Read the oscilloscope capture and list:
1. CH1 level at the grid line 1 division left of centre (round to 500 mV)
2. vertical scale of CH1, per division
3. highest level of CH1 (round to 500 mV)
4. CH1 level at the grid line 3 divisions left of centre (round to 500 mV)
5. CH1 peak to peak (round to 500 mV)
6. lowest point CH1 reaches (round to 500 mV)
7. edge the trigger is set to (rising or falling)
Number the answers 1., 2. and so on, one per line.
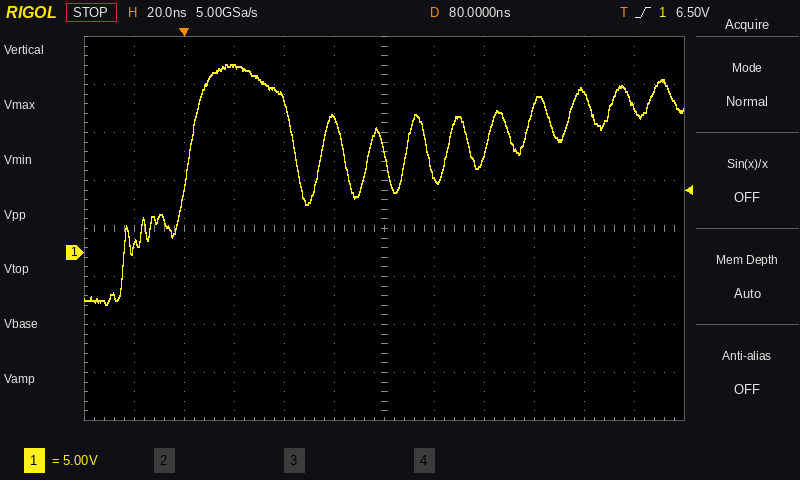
1. 14.0 V
2. 5 V
3. 19.5 V
4. 19.5 V
5. 25.0 V
6. -5.5 V
7. rising
